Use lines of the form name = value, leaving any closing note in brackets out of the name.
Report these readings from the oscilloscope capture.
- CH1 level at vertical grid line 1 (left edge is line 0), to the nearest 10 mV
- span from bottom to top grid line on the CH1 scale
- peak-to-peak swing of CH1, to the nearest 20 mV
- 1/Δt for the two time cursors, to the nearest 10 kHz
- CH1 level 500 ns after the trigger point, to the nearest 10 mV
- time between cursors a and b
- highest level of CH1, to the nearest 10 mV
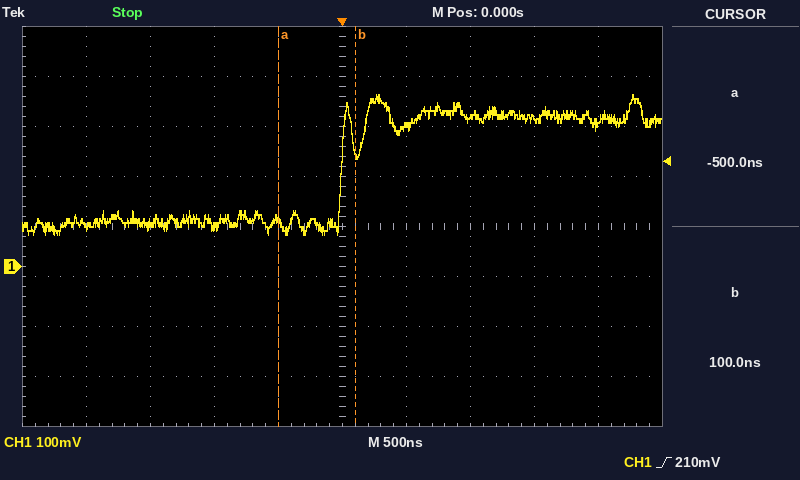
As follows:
CH1 level at vertical grid line 1 (left edge is line 0), to the nearest 10 mV = 80 mV
span from bottom to top grid line on the CH1 scale = 800 mV
peak-to-peak swing of CH1, to the nearest 20 mV = 280 mV
1/Δt for the two time cursors, to the nearest 10 kHz = 1.67 MHz
CH1 level 500 ns after the trigger point, to the nearest 10 mV = 280 mV
time between cursors a and b = 600 ns
highest level of CH1, to the nearest 10 mV = 340 mV
